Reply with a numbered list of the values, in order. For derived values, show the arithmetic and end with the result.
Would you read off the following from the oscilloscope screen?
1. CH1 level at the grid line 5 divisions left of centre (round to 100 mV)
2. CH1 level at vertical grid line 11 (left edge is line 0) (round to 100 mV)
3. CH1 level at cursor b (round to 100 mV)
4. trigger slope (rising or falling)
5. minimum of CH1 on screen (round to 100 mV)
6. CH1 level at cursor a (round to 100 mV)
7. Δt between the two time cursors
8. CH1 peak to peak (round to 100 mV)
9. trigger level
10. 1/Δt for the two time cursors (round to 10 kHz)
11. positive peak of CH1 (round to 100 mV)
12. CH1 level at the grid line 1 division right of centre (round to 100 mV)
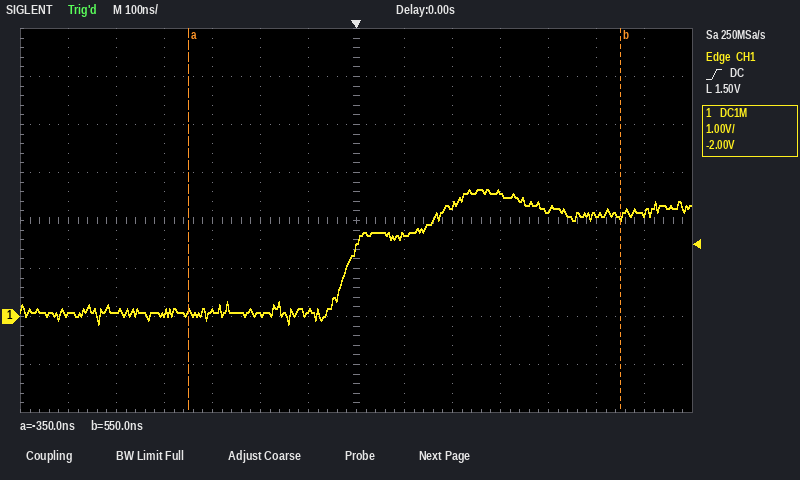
1. 100 mV
2. 2.2 V
3. 2.1 V
4. rising
5. -200 mV
6. 100 mV
7. 550 ns − (-350 ns) = 900 ns
8. 2.6 V − (-200 mV) = 2.8 V
9. 1.50 V
10. 1 / 900 ns ≈ 1.11 MHz
11. 2.6 V
12. 1.7 V
